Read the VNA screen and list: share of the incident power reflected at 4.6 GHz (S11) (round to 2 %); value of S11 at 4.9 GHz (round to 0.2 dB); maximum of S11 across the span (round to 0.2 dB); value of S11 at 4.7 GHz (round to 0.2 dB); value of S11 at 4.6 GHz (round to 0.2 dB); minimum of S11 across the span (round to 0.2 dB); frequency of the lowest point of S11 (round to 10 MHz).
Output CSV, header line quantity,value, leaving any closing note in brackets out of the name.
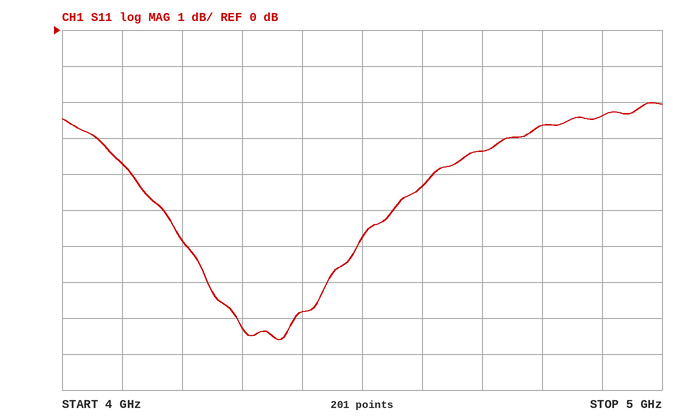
quantity,value
share of the incident power reflected at 4.6 GHz (S11),36 %
value of S11 at 4.9 GHz,-2.4 dB
maximum of S11 across the span,-2.0 dB
value of S11 at 4.7 GHz,-3.4 dB
value of S11 at 4.6 GHz,-4.4 dB
minimum of S11 across the span,-8.6 dB
frequency of the lowest point of S11,4.36 GHz
